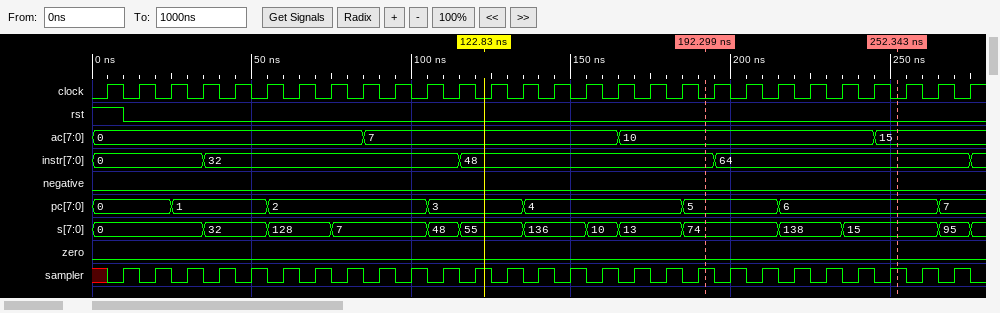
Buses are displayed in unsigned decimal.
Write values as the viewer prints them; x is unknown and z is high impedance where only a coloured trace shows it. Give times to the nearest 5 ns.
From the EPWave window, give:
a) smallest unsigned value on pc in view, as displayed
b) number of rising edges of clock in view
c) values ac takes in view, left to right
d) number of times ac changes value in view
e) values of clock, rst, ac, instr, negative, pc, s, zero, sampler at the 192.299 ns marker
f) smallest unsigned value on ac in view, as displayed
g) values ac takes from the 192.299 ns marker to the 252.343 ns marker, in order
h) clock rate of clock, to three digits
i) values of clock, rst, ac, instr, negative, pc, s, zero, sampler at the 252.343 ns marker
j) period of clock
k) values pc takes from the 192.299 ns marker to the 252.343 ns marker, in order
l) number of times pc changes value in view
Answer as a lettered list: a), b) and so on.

a) 0
b) 28
c) 0, 7, 10, 15
d) 3
e) clock=0, rst=0, ac=10, instr=48, negative=0, pc=5, s=74, zero=0, sampler=1
f) 0
g) 10, 15
h) 100 MHz
i) clock=0, rst=0, ac=15, instr=64, negative=0, pc=6, s=15, zero=0, sampler=1
j) 10 ns
k) 5, 6
l) 7
